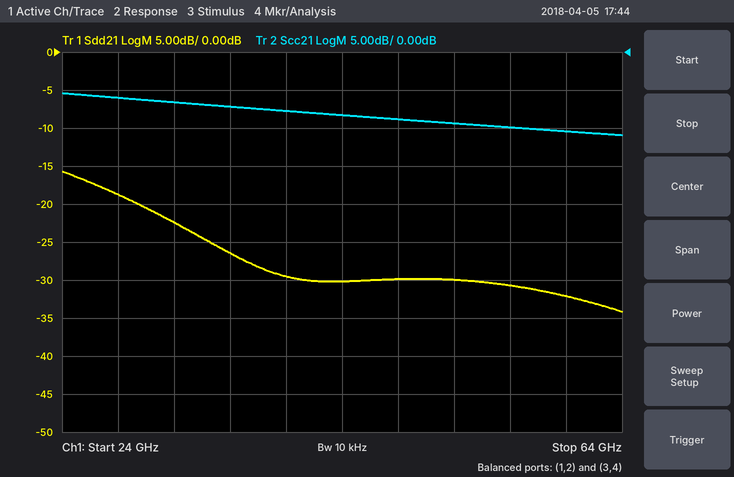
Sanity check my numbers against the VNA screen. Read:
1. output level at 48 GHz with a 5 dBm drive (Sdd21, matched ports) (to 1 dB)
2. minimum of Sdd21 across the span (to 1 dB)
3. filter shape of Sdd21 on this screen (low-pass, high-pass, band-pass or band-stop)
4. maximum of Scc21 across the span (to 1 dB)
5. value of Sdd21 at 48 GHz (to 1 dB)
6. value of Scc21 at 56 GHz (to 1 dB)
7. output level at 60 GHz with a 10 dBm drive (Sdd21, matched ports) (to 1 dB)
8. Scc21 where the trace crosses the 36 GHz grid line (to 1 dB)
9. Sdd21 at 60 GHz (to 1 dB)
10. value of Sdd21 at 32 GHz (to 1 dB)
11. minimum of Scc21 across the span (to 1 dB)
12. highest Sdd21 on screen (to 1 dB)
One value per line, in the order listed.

-25 dBm
-34 dB
low-pass
-5 dB
-30 dB
-10 dB
-22 dBm
-7 dB
-32 dB
-22 dB
-11 dB
-16 dB
